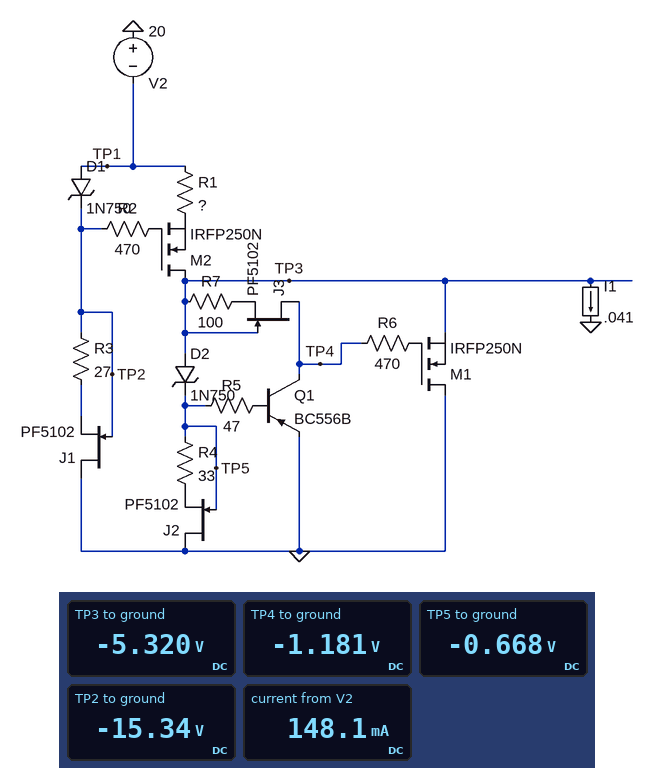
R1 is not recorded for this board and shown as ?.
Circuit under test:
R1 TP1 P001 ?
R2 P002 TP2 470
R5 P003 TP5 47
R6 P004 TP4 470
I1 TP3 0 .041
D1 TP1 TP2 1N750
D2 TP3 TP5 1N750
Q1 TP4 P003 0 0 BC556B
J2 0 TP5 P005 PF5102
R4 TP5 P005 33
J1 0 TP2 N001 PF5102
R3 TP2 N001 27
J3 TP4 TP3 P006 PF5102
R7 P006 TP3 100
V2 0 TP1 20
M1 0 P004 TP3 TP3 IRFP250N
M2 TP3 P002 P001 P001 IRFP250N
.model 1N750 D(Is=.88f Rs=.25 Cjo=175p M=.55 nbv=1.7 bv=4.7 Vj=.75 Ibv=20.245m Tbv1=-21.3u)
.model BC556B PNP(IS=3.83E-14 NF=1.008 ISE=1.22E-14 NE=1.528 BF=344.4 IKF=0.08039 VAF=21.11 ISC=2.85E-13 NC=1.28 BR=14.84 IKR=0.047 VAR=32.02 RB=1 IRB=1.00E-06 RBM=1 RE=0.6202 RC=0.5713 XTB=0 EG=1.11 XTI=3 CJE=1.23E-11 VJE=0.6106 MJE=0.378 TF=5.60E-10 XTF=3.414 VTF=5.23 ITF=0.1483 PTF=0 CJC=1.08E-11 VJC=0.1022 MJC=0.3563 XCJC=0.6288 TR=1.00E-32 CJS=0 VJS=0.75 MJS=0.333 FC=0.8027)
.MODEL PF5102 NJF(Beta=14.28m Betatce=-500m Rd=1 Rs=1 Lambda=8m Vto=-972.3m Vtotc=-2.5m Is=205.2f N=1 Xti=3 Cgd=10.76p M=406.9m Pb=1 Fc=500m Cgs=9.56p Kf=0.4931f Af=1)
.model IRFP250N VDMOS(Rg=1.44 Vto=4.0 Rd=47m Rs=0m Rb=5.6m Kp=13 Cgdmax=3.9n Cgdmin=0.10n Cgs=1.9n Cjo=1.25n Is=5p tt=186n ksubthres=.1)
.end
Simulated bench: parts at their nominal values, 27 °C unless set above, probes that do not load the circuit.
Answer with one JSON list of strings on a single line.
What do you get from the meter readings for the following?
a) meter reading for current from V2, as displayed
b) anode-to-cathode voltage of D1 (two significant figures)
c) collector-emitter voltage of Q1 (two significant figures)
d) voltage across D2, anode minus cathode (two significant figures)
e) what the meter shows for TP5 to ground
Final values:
["148.1 mA", "-4.7 V", "-1.2 V", "-4.7 V", "-0.668 V"]
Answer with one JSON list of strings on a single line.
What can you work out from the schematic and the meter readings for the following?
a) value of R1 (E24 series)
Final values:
["3.9 Ω"]
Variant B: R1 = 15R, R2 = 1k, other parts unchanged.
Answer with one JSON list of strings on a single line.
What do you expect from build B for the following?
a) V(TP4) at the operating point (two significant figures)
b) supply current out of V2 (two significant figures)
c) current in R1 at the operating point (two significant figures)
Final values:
["-1.3 V", "51 mA", "43 mA"]
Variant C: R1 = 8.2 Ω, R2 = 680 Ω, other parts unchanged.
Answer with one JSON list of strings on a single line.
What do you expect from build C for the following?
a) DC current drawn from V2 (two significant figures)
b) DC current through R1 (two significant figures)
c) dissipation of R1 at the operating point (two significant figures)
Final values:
["82 mA", "73 mA", "44 mW"]
